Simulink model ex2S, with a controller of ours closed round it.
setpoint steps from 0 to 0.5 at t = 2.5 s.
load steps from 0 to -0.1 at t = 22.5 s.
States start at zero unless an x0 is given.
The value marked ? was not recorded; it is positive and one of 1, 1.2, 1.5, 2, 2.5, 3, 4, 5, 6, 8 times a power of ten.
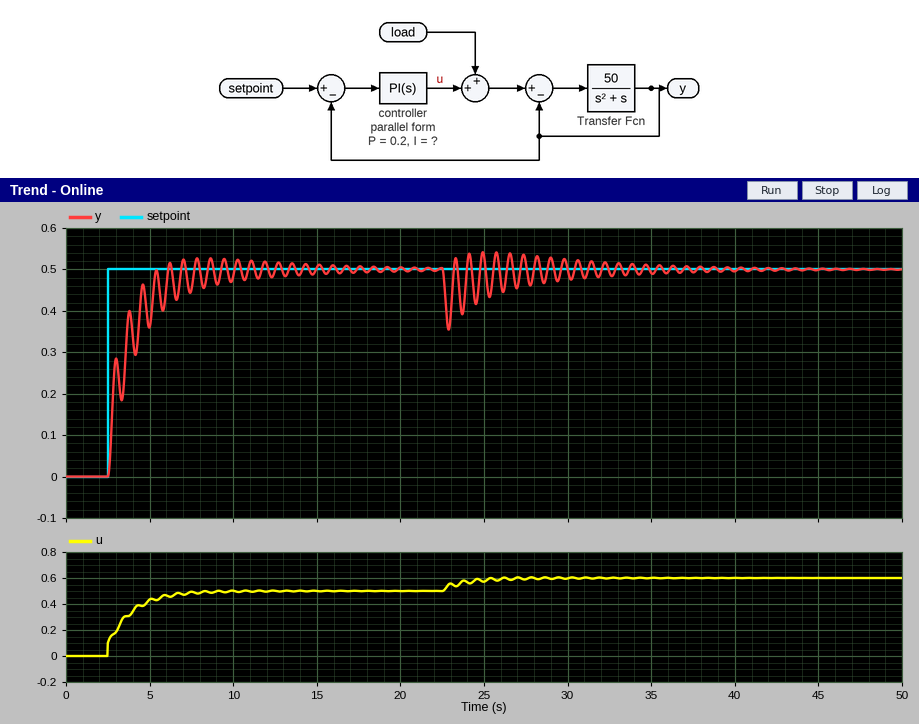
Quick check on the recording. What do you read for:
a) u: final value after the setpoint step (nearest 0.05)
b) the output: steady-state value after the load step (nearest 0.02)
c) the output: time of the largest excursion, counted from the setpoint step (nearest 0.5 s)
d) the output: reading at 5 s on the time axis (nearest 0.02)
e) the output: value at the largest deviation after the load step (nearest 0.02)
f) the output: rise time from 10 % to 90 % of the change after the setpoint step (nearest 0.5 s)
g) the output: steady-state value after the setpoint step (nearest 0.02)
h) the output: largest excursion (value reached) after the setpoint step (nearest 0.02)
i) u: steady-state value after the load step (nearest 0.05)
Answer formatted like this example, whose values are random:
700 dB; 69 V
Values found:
0.50; 0.50; 6.0 s; 0.36; 0.36; 2.0 s; 0.50; 0.52; 0.60
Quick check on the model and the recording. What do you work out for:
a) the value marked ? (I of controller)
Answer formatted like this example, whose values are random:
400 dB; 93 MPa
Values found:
0.8
